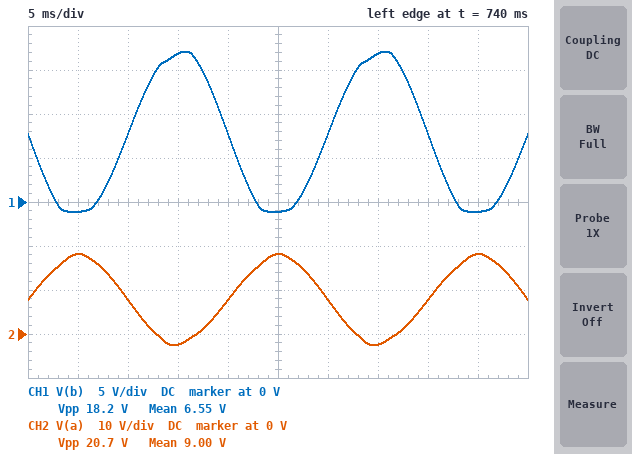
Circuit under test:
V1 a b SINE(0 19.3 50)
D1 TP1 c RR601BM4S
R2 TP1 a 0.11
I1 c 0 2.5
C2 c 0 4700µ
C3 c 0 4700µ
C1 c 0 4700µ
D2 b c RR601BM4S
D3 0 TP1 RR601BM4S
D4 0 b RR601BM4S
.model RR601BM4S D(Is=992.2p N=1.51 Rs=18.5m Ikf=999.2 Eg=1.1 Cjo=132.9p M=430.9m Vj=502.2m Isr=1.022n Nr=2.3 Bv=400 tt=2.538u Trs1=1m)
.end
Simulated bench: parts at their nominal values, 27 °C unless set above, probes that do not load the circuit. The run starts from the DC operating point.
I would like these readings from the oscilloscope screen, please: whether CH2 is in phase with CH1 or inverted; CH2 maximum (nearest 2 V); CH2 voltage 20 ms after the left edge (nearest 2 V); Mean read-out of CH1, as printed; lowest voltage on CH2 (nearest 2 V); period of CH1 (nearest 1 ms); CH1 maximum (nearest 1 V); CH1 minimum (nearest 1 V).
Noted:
inverted
18 V
8 V
6.55 V
-2 V
20 ms
17 V
-1 V
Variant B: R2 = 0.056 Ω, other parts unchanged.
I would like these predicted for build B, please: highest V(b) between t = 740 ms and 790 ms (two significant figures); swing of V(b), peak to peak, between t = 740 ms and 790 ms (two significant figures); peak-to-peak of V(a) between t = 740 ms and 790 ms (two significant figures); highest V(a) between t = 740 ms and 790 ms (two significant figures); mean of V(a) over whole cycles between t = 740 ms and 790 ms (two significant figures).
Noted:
18 V
19 V
20 V
18 V
8.0 V
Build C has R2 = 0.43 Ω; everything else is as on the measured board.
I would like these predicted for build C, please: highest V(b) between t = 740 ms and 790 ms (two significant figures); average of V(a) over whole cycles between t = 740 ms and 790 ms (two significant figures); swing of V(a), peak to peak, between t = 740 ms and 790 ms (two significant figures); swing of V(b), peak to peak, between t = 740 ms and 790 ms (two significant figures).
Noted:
15 V
6.7 V
23 V
16 V
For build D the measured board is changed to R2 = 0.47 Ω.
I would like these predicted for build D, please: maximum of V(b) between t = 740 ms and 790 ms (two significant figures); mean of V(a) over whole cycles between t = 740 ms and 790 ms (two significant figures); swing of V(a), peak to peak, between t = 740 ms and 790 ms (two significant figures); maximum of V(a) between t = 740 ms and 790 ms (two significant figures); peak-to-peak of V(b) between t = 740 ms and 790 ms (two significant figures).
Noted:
15 V
6.6 V
23 V
18 V
16 V
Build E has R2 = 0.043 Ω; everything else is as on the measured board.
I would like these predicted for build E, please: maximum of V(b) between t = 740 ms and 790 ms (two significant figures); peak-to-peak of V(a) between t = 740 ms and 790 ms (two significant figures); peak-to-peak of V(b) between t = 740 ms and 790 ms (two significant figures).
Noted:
18 V
20 V
19 V
